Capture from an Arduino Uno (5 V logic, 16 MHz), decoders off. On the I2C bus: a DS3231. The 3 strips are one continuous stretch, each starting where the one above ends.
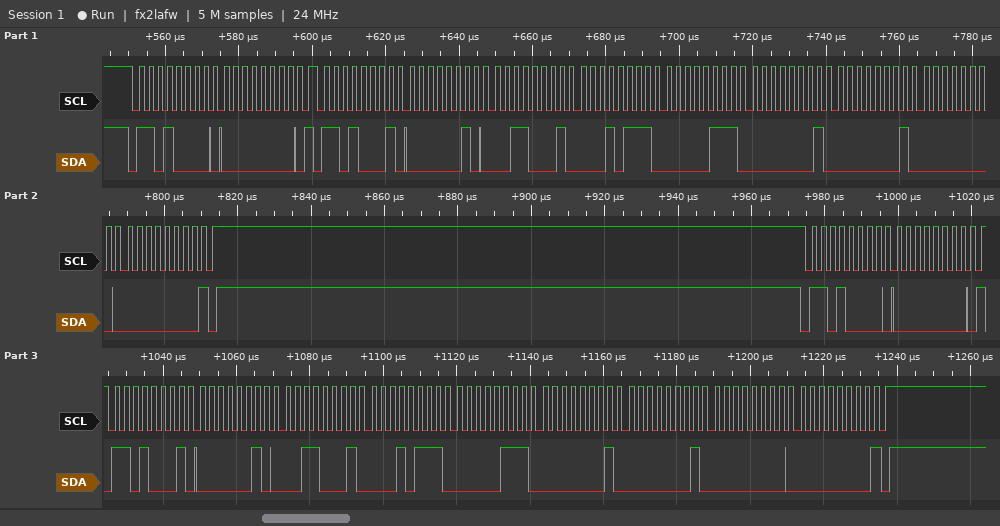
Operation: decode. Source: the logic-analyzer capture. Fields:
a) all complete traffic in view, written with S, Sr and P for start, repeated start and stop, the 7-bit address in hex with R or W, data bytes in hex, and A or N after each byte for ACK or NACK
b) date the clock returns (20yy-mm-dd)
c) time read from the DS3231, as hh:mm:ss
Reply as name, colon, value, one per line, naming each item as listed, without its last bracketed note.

all complete traffic in view, written with S, Sr and P for start, repeated start and stop, the 7-bit address in hex with R or W, data bytes in hex, and A or N after each byte for ACK or NACK: S 68W A 00 A Sr 68R A 02 A 31 A 17 A 07 A 01 A 01 A 00 A 00 N P S 68W A 00 A Sr 68R A 02 A 31 A 17 A 07 A 01 A 01 A 00 A 00 N P
date the clock returns: 2000-01-01
time read from the DS3231, as hh:mm:ss: 17:31:02
